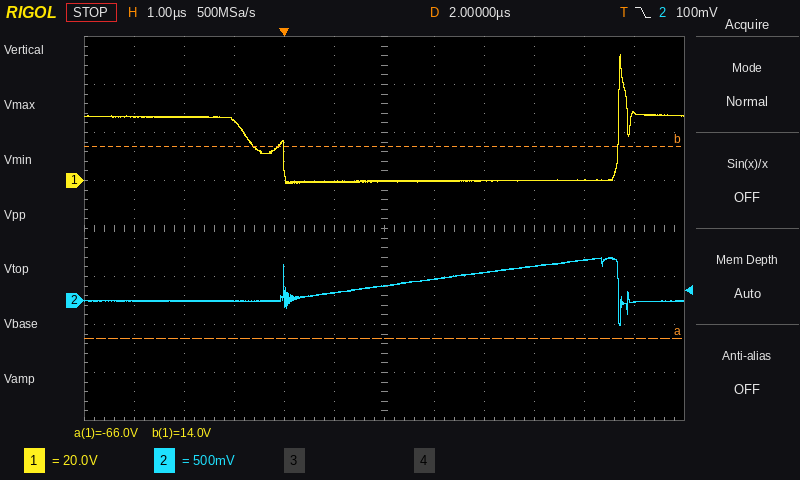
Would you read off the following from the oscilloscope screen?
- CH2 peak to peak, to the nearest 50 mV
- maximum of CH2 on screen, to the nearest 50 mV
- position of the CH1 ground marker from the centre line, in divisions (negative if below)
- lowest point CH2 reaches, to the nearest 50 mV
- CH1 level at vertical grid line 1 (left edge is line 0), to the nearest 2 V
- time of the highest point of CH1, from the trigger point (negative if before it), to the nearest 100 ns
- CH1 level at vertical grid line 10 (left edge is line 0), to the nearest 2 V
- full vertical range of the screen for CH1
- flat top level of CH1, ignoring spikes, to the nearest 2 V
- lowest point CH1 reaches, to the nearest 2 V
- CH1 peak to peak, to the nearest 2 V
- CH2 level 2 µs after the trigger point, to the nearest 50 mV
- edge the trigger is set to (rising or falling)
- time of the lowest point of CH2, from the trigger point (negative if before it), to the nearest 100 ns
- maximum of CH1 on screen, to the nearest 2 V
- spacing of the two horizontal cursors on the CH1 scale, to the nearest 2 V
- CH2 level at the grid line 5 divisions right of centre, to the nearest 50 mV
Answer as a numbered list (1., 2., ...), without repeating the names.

1. 700 mV
2. 450 mV
3. +1.0 div
4. -250 mV
5. 26 V
6. +6.7 µs
7. 0 V
8. 160 V
9. 26 V
10. -2 V
11. 54 V
12. 150 mV
13. falling
14. +6.7 µs
15. 52 V
16. 80 V
17. 0 mV
